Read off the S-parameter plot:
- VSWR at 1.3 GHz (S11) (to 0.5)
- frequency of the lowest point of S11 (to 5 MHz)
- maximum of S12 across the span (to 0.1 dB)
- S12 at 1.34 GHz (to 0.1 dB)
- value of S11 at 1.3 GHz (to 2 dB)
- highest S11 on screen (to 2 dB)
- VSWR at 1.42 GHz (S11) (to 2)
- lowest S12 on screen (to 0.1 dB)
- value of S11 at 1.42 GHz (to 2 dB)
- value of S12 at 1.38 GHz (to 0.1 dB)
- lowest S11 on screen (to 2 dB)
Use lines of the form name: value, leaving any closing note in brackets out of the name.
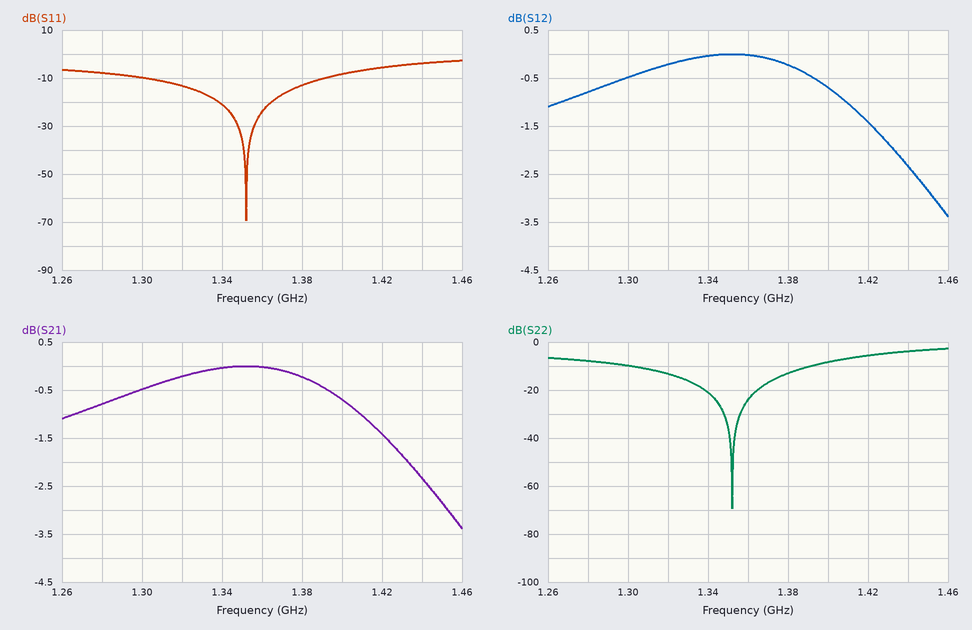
VSWR at 1.3 GHz (S11): 2.0
frequency of the lowest point of S11: 1.350 GHz
maximum of S12 across the span: 0.0 dB
S12 at 1.34 GHz: 0.0 dB
value of S11 at 1.3 GHz: -10 dB
highest S11 on screen: -2 dB
VSWR at 1.42 GHz (S11): 4
lowest S12 on screen: -3.4 dB
value of S11 at 1.42 GHz: -6 dB
value of S12 at 1.38 GHz: -0.2 dB
lowest S11 on screen: -70 dB
